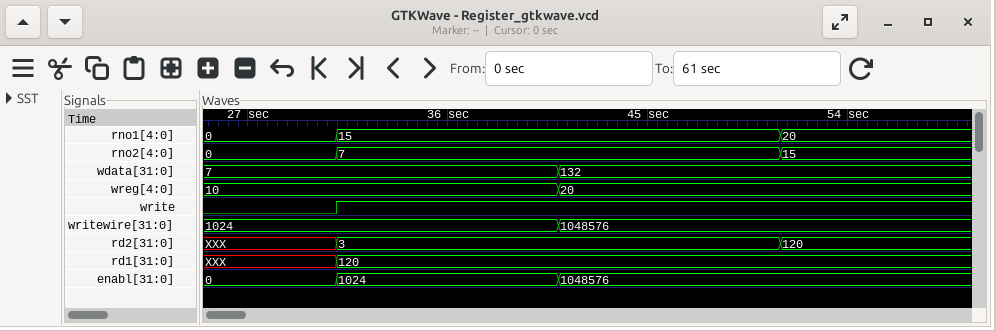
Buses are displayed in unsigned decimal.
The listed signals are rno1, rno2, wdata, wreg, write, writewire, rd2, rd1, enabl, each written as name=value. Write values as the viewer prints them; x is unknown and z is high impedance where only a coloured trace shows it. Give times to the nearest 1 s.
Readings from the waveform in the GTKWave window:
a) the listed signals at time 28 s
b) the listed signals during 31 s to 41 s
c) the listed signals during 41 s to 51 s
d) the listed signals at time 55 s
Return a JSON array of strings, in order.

["rno1=0, rno2=0, wdata=7, wreg=10, write=0, writewire=1024, rd2=XXX, rd1=XXX, enabl=0", "rno1=15, rno2=7, wdata=7, wreg=10, write=1, writewire=1024, rd2=3, rd1=120, enabl=1024", "rno1=15, rno2=7, wdata=132, wreg=20, write=1, writewire=1048576, rd2=3, rd1=120, enabl=1048576", "rno1=20, rno2=15, wdata=132, wreg=20, write=1, writewire=1048576, rd2=120, rd1=120, enabl=1048576"]
